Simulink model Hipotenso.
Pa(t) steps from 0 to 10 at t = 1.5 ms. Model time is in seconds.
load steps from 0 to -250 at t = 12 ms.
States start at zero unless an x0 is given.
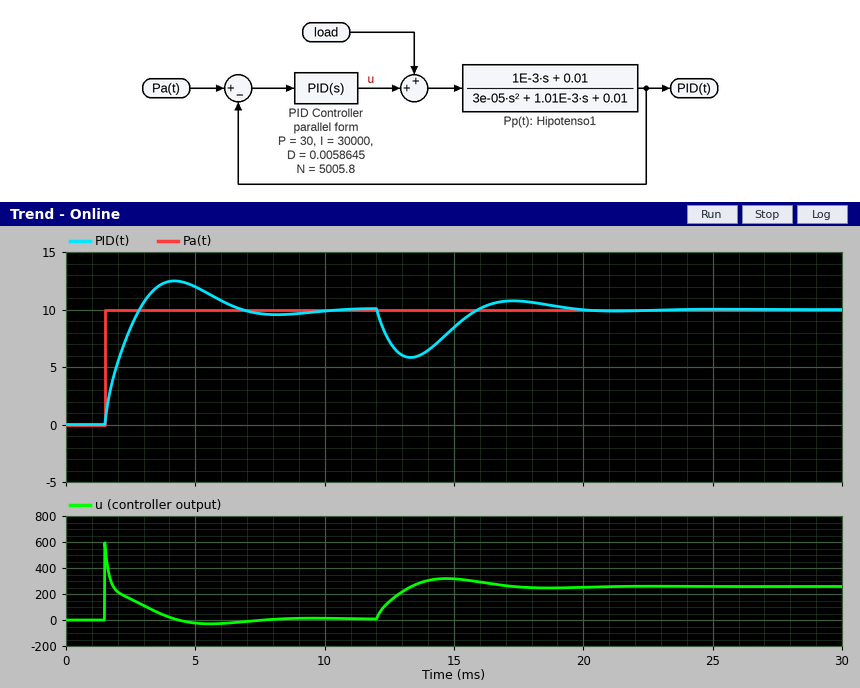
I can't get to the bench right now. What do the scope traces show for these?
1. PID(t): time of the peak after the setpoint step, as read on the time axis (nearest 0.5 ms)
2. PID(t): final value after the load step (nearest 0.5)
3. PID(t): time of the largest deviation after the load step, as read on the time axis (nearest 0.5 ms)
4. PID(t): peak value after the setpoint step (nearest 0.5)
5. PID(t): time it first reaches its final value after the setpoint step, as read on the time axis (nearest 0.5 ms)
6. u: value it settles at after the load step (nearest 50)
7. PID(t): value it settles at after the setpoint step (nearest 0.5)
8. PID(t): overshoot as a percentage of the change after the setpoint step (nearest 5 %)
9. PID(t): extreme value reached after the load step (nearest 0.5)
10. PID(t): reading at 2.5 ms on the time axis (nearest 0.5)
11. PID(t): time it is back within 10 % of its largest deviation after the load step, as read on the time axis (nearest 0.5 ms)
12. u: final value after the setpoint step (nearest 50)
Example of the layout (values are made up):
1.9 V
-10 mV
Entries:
4.0 ms
10.0
13.5 ms
12.5
3.0 ms
250
10.0
25 %
6.0
8.5
18.5 ms
0
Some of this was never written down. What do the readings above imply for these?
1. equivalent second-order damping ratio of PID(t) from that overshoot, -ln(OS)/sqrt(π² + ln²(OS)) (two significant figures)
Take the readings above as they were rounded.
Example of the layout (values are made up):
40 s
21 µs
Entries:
0.40
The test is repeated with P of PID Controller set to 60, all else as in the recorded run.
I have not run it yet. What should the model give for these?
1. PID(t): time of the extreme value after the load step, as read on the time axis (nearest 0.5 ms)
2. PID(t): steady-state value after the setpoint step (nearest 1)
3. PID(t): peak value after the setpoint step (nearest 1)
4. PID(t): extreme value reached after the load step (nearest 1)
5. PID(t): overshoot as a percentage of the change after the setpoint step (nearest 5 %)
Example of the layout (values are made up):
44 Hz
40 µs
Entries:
13.0 ms
10
11
7
10 %
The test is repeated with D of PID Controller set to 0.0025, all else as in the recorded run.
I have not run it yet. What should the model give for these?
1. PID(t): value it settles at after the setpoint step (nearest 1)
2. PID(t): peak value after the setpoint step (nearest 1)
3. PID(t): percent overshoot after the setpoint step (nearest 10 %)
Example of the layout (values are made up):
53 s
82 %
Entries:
10
13
30 %
